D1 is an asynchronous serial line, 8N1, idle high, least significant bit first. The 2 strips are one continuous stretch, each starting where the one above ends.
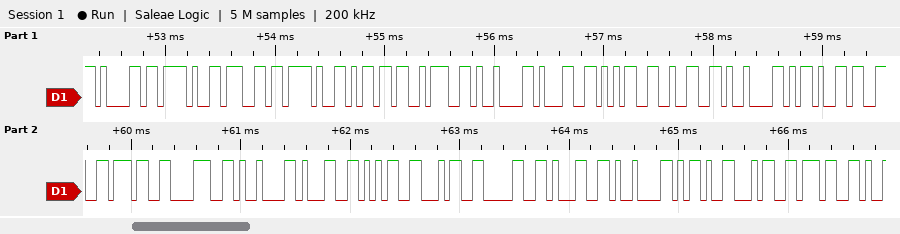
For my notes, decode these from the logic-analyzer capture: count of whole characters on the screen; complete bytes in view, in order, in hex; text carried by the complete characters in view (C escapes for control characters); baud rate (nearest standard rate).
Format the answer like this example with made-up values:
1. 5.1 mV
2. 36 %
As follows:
1. 25
2. 61 2F 67 2F 6D 3A 09 31 35 32 09 2D 33 37 38 09 31 35 34 30 31 09 2D 34 37
3. "a/g/m:\t152\t-378\t15401\t-47"
4. 19200 baud
